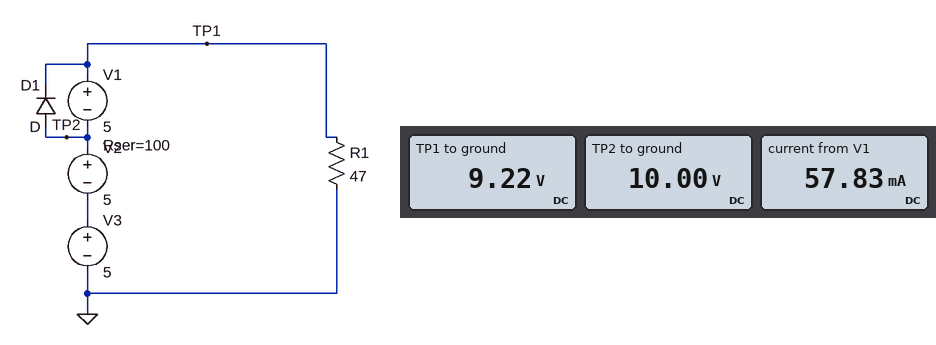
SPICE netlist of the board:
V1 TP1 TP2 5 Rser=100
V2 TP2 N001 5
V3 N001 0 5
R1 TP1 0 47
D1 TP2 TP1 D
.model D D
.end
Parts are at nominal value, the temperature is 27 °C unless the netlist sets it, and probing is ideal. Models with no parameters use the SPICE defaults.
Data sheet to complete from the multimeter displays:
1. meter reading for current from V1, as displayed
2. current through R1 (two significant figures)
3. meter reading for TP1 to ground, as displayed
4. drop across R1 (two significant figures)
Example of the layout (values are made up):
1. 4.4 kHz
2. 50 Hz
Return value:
1. 57.83 mA
2. 200 mA
3. 9.22 V
4. 9.2 V
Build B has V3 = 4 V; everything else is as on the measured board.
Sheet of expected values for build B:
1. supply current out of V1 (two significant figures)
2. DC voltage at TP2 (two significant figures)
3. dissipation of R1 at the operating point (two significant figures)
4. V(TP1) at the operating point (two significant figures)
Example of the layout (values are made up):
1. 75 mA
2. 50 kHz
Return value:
1. 58 mA
2. 9.0 V
3. 1.4 W
4. 8.2 V
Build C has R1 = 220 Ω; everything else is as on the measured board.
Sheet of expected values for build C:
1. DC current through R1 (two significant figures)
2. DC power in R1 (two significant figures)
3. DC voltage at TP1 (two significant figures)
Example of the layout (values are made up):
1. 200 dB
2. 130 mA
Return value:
1. 47 mA
2. 480 mW
3. 10 V
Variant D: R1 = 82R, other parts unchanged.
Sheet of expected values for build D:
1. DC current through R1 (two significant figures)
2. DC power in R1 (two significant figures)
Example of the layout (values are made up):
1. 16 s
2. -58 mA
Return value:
1. 110 mA
2. 1.0 W
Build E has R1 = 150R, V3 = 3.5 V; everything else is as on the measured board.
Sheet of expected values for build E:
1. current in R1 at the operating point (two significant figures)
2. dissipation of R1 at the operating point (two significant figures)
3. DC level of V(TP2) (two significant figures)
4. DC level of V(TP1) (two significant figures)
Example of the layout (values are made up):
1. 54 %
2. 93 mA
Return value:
1. 54 mA
2. 440 mW
3. 8.5 V
4. 8.1 V
